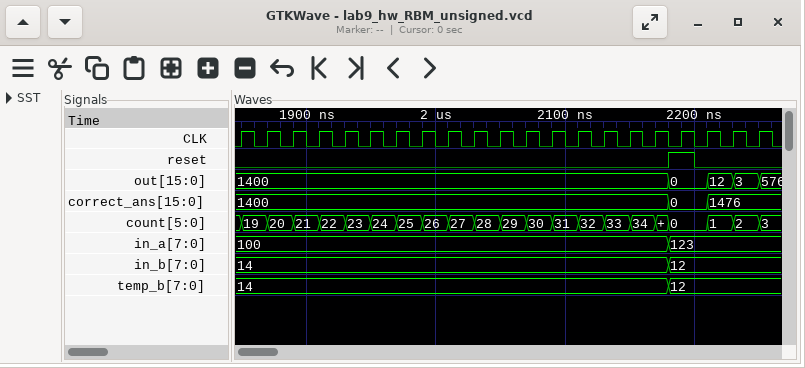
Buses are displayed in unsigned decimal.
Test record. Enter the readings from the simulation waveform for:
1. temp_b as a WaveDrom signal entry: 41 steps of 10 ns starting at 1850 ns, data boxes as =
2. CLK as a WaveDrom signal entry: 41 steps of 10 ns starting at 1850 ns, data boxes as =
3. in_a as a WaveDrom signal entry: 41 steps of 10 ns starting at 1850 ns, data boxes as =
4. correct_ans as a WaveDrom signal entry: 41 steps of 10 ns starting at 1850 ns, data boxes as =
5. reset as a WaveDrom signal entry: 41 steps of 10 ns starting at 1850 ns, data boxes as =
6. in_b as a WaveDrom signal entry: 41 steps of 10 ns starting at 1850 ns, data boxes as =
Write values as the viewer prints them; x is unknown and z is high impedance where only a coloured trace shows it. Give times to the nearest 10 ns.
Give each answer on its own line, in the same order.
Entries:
{name: 'temp_b', wave: '=................................=.......', data: '14 12'}
{name: 'CLK', wave: '10101010101010101010101010101010101010101'}
{name: 'in_a', wave: '=................................=.......', data: '100 123'}
{name: 'correct_ans', wave: '=................................=..=....', data: '1400 0 1476'}
{name: 'reset', wave: '0................................1.0.....'}
{name: 'in_b', wave: '=................................=.......', data: '14 12'}
